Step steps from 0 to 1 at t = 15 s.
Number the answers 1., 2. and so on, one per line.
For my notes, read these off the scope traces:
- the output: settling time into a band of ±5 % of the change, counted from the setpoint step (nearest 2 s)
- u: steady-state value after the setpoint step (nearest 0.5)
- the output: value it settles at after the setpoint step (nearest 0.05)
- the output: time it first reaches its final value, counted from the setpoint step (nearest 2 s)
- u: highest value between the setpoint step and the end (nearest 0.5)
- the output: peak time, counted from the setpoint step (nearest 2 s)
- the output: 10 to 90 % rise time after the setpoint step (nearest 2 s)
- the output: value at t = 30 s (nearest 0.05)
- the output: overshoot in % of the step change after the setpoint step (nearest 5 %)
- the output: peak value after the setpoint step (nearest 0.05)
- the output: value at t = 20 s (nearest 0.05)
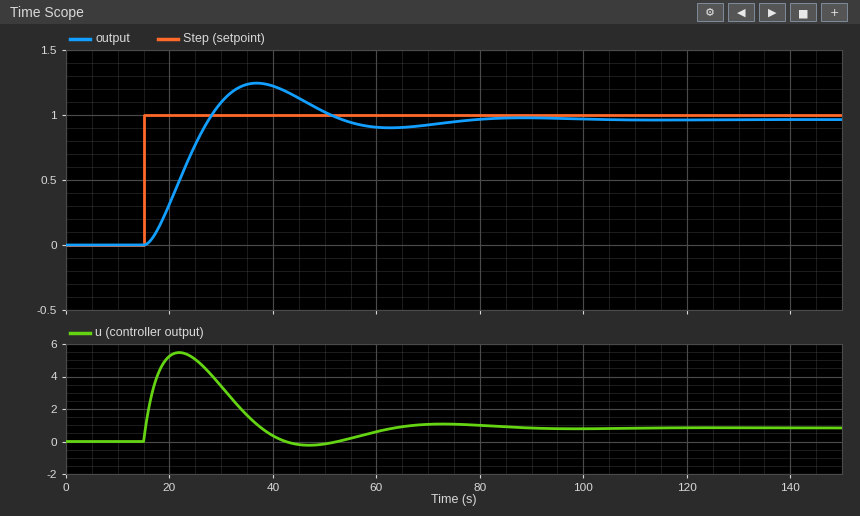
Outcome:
1. 54 s
2. 1.0
3. 0.95
4. 12 s
5. 5.5
6. 22 s
7. 8 s
8. 1.10
9. 30 %
10. 1.25
11. 0.30
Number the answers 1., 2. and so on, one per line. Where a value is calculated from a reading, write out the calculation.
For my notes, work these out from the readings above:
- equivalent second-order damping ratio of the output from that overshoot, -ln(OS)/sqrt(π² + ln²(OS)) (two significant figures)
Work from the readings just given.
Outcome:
1. ln(0.3) = -1.204; 1.204 / sqrt(9.870 + 1.450) = 0.36
